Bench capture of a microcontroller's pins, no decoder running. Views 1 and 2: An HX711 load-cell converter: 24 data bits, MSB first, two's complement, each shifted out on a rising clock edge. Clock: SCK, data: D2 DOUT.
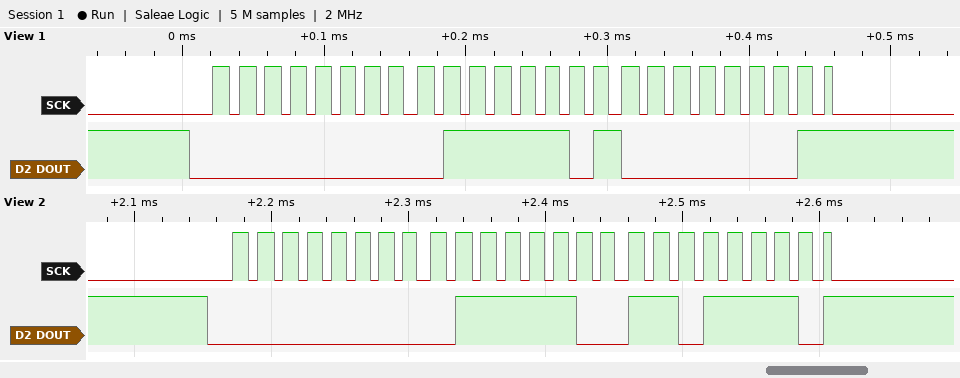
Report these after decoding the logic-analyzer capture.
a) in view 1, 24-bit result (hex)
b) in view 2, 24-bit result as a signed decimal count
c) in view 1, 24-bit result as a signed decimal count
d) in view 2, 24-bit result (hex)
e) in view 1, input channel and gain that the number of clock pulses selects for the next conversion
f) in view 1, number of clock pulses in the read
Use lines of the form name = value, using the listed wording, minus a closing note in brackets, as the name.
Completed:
in view 1, 24-bit result = 0x007D01
in view 2, 24-bit result as a signed decimal count = 31966
in view 1, 24-bit result as a signed decimal count = 32001
in view 2, 24-bit result = 0x007CDE
in view 1, input channel and gain that the number of clock pulses selects for the next conversion = channel A, gain 128
in view 1, number of clock pulses in the read = 25
